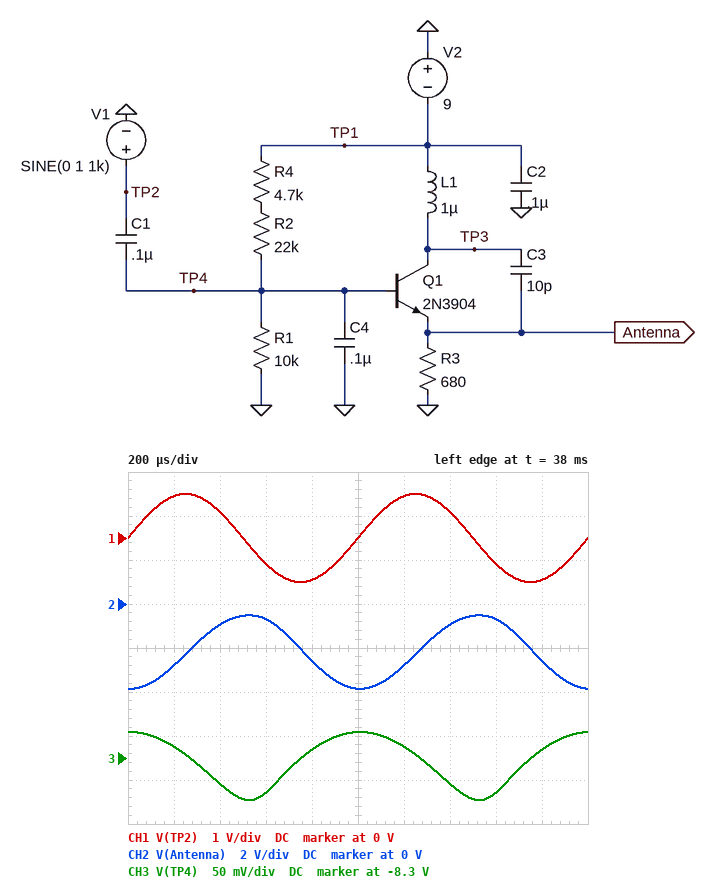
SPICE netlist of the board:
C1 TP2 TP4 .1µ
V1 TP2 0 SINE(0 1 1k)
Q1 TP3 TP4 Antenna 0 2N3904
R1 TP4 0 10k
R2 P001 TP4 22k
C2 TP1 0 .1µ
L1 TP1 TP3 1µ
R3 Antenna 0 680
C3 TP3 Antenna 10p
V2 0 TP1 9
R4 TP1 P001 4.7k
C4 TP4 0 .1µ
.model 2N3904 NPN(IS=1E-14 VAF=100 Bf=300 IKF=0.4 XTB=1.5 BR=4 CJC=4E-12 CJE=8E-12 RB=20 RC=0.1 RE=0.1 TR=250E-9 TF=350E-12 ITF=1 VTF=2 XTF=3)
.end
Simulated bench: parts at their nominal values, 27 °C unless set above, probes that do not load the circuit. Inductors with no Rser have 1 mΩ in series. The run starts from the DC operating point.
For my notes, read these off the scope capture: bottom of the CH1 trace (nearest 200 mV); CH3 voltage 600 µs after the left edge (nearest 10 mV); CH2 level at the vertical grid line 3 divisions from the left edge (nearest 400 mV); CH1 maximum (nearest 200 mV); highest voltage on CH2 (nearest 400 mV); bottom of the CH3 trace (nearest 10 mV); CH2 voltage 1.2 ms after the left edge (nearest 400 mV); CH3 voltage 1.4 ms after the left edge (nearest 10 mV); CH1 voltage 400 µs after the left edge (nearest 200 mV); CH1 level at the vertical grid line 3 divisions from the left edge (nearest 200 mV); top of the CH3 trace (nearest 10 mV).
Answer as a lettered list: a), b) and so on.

a) -1.0 V
b) -8.34 V
c) -800 mV
d) 1.0 V
e) -400 mV
f) -8.35 V
g) -2.8 V
h) -8.33 V
i) 600 mV
j) -600 mV
k) -8.27 V
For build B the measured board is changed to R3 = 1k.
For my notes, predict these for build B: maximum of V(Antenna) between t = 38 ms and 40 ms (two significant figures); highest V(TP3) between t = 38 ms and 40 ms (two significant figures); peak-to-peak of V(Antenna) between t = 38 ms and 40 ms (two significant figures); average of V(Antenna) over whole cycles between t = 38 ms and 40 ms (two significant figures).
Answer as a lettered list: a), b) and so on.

a) -760 mV
b) -9.0 V
c) 4.9 V
d) -3.2 V
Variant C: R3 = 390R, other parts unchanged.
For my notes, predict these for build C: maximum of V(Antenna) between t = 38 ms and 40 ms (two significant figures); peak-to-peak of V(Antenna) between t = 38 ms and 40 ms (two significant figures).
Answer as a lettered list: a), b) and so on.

a) -300 mV
b) 1.9 V
